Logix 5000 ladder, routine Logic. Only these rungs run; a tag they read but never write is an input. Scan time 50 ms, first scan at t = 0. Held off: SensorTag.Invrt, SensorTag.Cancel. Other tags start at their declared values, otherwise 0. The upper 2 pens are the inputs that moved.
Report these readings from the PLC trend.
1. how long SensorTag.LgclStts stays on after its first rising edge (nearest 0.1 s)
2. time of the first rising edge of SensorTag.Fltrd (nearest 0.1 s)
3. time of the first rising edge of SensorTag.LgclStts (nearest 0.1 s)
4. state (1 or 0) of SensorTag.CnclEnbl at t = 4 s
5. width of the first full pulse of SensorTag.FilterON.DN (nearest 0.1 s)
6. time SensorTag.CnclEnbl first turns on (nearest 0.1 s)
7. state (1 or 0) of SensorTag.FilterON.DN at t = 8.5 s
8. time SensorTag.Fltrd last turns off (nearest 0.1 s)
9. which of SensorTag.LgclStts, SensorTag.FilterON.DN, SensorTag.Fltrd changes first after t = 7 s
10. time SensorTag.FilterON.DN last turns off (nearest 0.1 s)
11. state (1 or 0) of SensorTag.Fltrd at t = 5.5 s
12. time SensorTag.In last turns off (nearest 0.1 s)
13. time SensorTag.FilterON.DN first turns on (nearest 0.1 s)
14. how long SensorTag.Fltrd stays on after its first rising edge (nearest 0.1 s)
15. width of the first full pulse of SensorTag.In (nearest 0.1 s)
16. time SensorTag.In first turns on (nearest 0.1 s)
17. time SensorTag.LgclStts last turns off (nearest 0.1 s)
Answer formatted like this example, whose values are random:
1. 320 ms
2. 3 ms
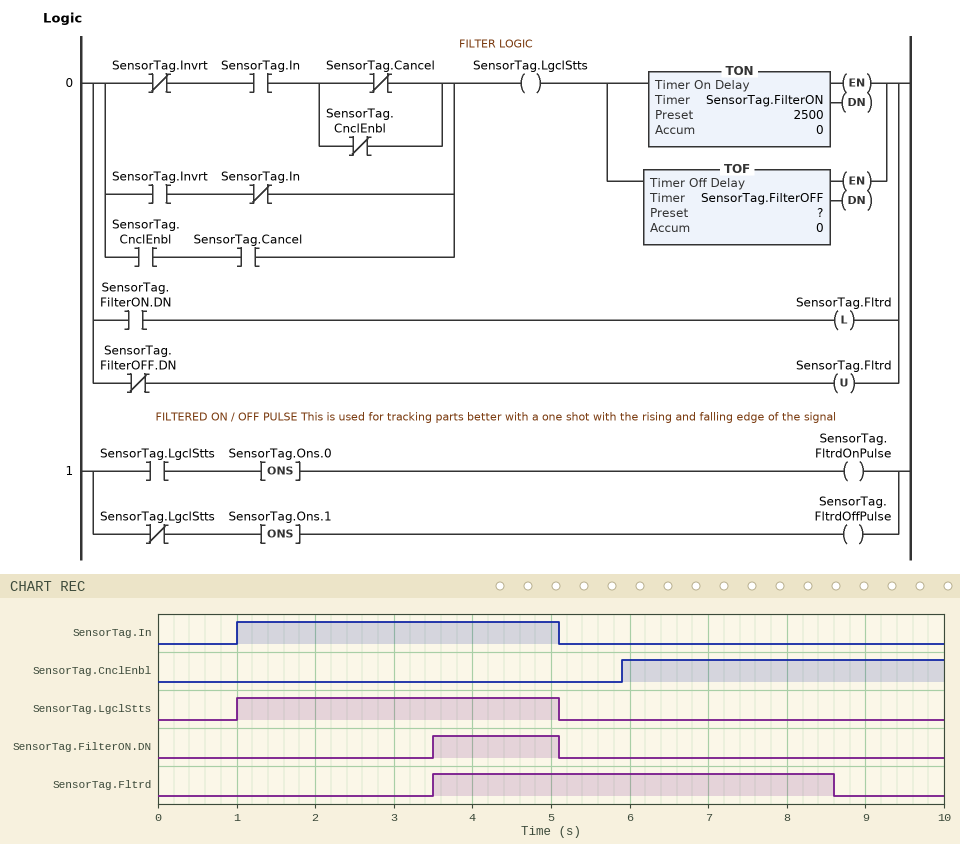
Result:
1. 4.1 s
2. 3.5 s
3. 1.0 s
4. 0
5. 1.6 s
6. 5.9 s
7. 0
8. 8.6 s
9. SensorTag.Fltrd
10. 5.1 s
11. 1
12. 5.1 s
13. 3.5 s
14. 5.1 s
15. 4.1 s
16. 1.0 s
17. 5.1 s
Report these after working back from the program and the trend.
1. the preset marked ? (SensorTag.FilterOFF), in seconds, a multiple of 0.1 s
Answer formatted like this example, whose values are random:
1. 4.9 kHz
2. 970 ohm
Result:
1. 3.5 s
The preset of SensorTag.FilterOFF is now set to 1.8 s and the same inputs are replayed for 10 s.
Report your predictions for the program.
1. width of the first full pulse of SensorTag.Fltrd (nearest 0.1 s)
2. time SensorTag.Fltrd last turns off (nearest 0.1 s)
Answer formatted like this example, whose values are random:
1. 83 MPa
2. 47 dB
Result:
1. 3.4 s
2. 6.9 s
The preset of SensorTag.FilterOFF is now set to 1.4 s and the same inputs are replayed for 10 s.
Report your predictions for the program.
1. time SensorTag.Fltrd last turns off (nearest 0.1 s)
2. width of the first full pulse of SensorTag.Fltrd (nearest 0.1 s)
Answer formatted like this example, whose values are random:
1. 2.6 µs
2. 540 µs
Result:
1. 6.5 s
2. 3.0 s
